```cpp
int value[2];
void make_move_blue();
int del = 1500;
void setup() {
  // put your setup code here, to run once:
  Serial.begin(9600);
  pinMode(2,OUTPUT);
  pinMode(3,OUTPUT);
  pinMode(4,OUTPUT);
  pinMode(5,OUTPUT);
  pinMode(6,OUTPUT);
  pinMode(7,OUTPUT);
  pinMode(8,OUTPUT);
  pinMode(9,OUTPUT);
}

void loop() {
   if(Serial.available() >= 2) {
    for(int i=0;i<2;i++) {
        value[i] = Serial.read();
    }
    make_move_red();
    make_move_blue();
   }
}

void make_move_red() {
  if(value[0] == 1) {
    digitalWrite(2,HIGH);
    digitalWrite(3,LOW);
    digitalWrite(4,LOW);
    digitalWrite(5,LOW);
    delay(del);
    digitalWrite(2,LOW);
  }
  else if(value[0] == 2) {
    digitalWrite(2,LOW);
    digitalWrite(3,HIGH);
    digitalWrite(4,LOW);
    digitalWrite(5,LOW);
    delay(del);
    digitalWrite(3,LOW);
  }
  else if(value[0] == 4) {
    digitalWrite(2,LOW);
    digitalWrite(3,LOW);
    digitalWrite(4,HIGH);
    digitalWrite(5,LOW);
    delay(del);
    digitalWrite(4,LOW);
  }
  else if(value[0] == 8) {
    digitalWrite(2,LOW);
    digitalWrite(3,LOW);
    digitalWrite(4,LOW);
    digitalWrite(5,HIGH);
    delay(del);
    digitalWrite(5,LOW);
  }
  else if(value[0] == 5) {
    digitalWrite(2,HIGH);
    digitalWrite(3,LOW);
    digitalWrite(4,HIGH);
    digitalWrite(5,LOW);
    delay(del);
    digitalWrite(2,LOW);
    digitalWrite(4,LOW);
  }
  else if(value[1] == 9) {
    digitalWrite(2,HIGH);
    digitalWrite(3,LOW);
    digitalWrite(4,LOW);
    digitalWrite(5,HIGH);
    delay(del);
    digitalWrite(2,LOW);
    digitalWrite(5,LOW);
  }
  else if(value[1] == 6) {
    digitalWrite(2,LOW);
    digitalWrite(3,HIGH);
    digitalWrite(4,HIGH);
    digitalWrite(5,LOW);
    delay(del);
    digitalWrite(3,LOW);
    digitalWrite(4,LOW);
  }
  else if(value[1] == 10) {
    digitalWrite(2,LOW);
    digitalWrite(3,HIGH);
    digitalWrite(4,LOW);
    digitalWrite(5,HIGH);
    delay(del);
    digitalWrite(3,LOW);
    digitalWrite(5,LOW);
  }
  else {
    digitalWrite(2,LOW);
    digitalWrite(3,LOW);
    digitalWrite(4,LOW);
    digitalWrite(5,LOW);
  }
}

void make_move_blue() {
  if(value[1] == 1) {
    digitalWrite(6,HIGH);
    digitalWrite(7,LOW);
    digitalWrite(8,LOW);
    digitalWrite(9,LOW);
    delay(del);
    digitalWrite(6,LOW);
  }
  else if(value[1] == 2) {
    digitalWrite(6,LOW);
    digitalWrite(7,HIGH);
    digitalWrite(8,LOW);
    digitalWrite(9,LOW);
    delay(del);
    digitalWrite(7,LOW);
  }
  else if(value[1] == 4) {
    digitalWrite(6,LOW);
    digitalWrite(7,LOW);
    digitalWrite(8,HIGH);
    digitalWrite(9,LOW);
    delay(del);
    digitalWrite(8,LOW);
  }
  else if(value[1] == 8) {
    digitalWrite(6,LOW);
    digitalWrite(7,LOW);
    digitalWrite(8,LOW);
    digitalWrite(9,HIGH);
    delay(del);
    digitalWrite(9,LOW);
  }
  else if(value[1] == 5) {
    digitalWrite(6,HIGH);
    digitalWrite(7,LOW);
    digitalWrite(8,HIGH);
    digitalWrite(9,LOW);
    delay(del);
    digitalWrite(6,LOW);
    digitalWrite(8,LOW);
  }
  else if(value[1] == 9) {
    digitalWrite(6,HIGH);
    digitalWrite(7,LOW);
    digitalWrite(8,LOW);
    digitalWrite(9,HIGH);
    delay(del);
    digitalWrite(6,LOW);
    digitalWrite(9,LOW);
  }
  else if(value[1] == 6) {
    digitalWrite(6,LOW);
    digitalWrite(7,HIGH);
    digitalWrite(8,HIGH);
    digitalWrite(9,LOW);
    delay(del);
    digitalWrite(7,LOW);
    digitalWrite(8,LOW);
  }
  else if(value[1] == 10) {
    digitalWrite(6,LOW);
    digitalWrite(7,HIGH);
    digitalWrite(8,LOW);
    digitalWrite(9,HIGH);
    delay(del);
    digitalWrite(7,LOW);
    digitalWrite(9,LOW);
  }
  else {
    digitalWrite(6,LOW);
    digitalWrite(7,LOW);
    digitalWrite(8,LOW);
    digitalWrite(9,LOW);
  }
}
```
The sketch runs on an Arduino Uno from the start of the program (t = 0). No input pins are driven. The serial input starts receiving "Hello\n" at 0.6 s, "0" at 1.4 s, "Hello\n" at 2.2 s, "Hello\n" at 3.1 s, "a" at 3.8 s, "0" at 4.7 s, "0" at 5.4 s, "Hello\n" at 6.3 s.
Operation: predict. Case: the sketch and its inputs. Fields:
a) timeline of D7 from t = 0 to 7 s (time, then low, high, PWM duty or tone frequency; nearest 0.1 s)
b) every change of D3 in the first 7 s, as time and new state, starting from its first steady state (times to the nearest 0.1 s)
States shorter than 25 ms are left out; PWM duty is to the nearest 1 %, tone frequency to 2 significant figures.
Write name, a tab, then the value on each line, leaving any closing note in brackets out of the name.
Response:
timeline of D7 from t = 0 to 7 s	0 s low; 2.1 s high; 3.6 s low
every change of D3 in the first 7 s, as time and new state, starting from its first steady state	0 s low; 0.6 s high; 2.1 s low; 6.3 s high
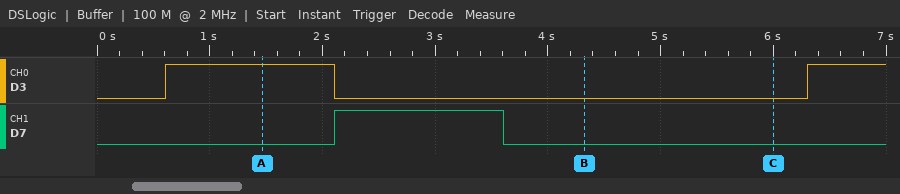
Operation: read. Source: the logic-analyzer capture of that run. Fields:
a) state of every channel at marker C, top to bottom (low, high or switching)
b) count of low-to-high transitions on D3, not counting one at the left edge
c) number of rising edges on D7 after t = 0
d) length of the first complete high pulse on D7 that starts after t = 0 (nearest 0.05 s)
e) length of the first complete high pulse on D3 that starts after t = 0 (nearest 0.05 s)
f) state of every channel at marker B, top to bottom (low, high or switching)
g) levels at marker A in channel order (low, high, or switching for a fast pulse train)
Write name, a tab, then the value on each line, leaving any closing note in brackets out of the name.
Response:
state of every channel at marker C, top to bottom	D3 low, D7 low
count of low-to-high transitions on D3, not counting one at the left edge	2
number of rising edges on D7 after t = 0	1
length of the first complete high pulse on D7 that starts after t = 0	1.50 s
length of the first complete high pulse on D3 that starts after t = 0	1.50 s
state of every channel at marker B, top to bottom	D3 low, D7 low
levels at marker A in channel order	D3 high, D7 low
